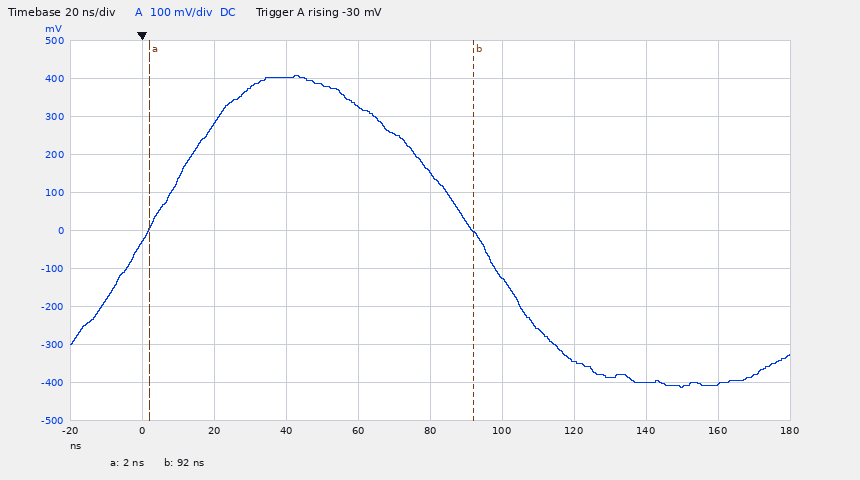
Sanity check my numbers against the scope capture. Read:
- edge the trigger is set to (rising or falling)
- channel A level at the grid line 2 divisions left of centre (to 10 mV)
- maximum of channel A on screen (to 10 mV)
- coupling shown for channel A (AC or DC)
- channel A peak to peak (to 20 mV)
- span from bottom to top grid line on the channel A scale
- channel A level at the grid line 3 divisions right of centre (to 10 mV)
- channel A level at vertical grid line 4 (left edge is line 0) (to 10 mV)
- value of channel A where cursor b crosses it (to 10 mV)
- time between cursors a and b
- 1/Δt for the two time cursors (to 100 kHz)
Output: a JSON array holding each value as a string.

["rising", "400 mV", "410 mV", "DC", "820 mV", "1 V", "-400 mV", "330 mV", "0 mV", "90 ns", "11.1 MHz"]
